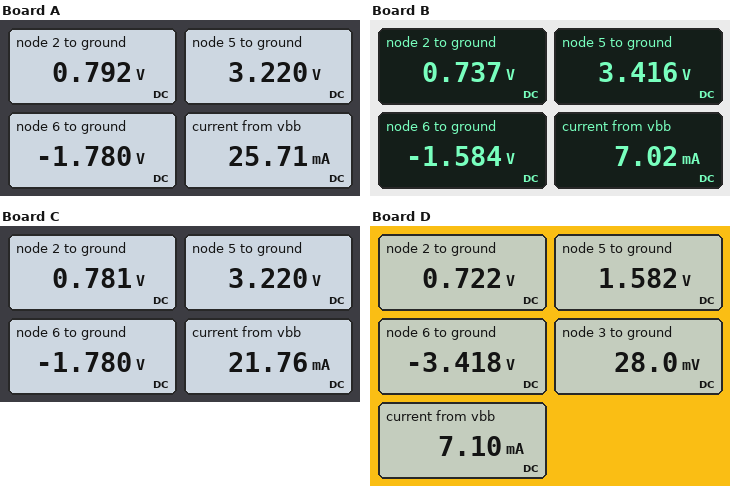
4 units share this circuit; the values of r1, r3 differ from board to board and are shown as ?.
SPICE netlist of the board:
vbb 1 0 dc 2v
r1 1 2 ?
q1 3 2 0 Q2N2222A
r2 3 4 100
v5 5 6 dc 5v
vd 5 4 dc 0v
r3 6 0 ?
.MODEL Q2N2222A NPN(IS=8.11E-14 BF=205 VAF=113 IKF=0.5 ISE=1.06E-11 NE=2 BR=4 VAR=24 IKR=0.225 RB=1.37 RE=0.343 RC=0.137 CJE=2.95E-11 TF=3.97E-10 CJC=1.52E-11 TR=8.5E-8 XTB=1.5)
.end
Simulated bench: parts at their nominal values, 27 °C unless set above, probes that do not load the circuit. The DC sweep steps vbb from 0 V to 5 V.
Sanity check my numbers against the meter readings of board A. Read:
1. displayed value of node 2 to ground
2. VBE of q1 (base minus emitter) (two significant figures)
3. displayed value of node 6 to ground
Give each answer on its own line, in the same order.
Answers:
0.792 V
790 mV
-1.780 V
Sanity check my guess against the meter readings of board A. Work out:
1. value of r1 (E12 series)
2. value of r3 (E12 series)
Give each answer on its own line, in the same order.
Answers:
47 Ω
56 Ω
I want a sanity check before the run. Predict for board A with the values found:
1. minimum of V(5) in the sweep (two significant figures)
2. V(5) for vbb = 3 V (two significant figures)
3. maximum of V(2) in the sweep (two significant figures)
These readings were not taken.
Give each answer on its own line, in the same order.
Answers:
3.2 V
3.2 V
930 mV
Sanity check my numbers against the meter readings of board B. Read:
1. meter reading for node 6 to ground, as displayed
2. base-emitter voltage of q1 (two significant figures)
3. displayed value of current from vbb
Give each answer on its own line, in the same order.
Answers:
-1.584 V
740 mV
7.02 mA
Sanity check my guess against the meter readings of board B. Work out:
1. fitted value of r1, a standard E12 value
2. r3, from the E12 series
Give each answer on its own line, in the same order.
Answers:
180 Ω
47 Ω
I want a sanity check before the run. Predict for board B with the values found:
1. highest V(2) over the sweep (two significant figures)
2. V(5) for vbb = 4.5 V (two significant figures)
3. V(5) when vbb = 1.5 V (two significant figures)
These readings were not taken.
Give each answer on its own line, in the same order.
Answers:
790 mV
3.4 V
3.4 V
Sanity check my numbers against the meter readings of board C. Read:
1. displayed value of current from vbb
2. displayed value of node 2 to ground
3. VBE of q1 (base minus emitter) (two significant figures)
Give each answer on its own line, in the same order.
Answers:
21.76 mA
0.781 V
780 mV
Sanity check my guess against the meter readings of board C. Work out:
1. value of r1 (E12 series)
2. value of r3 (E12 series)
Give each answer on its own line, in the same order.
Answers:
56 Ω
56 Ω
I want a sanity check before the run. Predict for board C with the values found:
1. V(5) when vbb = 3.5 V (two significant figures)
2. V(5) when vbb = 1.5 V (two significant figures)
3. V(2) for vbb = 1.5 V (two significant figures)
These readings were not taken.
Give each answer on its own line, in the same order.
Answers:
3.2 V
3.2 V
760 mV
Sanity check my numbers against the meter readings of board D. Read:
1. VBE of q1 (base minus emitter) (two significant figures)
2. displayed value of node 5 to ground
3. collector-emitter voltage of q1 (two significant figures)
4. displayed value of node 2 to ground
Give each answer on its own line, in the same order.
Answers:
720 mV
1.582 V
28 mV
0.722 V
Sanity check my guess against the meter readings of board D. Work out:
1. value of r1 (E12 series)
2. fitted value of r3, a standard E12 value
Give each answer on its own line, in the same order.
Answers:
180 Ω
220 Ω
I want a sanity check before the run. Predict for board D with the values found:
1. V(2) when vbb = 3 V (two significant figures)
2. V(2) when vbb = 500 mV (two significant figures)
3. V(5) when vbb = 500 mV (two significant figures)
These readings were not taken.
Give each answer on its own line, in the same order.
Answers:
740 mV
500 mV
5.0 V
